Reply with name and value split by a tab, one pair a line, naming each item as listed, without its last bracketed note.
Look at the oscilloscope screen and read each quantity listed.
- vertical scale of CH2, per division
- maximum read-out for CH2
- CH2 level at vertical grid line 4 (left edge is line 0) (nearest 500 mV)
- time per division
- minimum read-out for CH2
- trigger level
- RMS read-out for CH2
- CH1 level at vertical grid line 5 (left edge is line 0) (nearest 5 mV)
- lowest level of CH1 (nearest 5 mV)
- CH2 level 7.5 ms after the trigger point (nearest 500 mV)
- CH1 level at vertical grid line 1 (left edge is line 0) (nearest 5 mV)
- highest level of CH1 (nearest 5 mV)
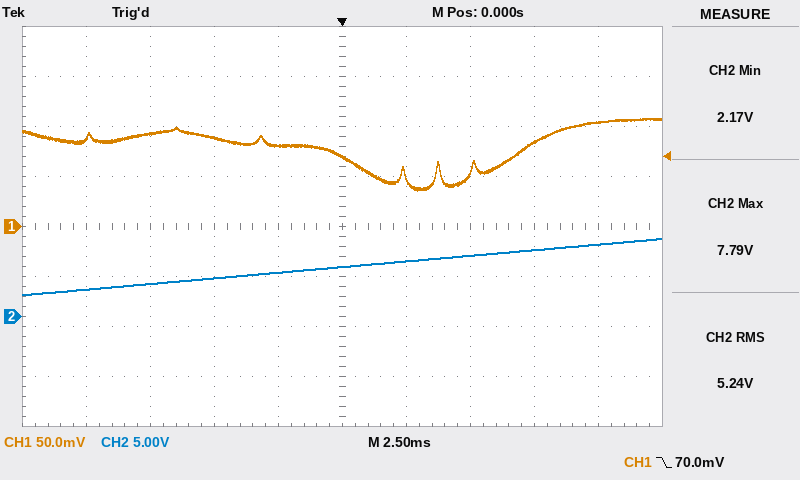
vertical scale of CH2, per division	5 V
maximum read-out for CH2	7.79 V
CH2 level at vertical grid line 4 (left edge is line 0)	4.5 V
time per division	2.5 ms
minimum read-out for CH2	2.17 V
trigger level	70.0 mV
RMS read-out for CH2	5.24 V
CH1 level at vertical grid line 5 (left edge is line 0)	70 mV
lowest level of CH1	35 mV
CH2 level 7.5 ms after the trigger point	6.5 V
CH1 level at vertical grid line 1 (left edge is line 0)	90 mV
highest level of CH1	110 mV
